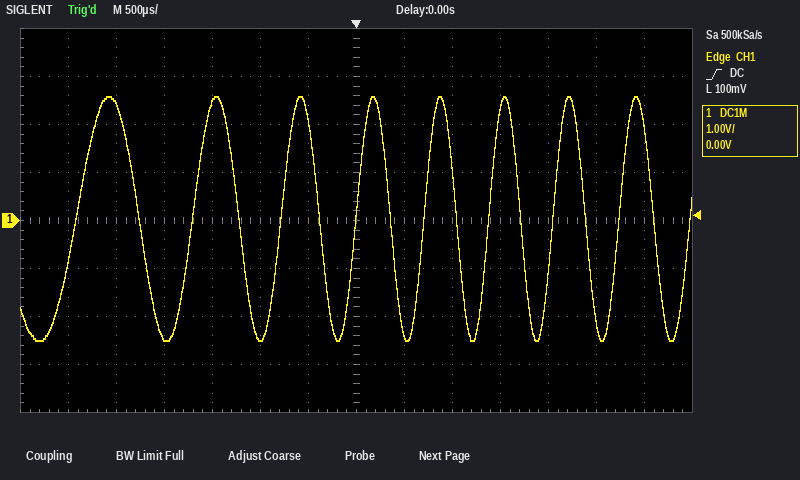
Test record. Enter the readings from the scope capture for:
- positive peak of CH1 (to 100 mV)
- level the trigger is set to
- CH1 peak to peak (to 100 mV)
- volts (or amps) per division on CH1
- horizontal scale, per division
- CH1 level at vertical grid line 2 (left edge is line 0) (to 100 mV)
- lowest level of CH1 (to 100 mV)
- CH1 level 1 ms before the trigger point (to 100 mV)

2.6 V
100 mV
5.1 V
1 V
500 µs
2.4 V
-2.5 V
-2.5 V
